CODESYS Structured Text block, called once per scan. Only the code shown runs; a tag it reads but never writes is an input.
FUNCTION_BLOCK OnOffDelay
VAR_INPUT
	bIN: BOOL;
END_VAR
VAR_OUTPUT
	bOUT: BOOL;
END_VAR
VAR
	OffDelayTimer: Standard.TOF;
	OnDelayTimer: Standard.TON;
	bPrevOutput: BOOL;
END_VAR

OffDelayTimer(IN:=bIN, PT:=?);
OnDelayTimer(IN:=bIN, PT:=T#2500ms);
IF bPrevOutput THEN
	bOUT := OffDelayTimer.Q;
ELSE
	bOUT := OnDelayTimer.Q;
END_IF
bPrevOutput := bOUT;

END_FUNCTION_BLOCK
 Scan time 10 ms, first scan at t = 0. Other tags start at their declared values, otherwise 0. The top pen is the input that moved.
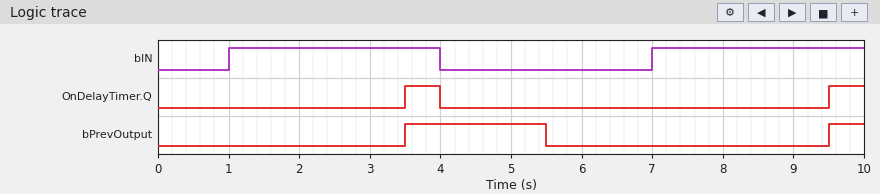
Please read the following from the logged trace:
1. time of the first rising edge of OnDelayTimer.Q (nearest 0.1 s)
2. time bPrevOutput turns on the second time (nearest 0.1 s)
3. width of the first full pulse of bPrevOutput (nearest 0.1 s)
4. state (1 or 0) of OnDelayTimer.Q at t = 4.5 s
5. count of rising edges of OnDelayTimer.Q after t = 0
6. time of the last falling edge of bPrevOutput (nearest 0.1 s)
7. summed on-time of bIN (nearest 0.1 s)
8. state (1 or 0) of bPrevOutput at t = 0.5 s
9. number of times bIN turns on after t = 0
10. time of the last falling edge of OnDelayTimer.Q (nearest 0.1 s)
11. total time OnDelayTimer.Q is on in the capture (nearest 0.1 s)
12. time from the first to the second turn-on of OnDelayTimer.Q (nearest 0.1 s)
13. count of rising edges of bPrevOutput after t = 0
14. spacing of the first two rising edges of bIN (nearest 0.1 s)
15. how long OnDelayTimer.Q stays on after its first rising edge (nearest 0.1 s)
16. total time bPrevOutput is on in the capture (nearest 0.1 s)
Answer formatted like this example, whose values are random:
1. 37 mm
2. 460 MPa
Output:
1. 3.5 s
2. 9.5 s
3. 2.0 s
4. 0
5. 2
6. 5.5 s
7. 6.0 s
8. 0
9. 2
10. 4.0 s
11. 1.0 s
12. 6.0 s
13. 2
14. 6.0 s
15. 0.5 s
16. 2.5 s
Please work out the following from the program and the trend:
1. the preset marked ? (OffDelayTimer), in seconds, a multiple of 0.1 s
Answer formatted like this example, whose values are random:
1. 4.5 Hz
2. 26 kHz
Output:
1. 1.5 s
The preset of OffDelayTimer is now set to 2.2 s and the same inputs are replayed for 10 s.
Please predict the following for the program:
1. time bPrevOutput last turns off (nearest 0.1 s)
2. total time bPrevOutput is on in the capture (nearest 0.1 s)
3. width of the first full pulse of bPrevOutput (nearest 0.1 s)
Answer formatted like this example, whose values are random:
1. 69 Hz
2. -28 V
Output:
1. 6.2 s
2. 3.2 s
3. 2.7 s
